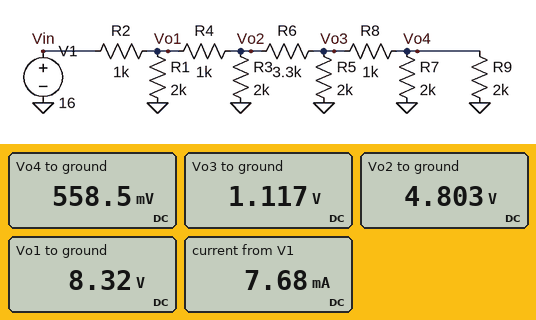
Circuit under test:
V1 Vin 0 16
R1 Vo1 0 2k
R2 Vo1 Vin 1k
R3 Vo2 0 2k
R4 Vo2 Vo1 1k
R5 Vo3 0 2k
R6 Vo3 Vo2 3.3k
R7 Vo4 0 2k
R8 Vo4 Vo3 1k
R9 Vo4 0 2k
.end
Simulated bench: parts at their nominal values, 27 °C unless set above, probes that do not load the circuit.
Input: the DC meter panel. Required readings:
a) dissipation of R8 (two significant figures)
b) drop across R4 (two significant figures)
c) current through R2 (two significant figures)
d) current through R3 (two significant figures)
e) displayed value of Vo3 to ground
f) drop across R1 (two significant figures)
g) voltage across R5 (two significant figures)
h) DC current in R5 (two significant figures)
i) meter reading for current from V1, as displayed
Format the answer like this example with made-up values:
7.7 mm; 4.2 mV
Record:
310 µW; 3.5 V; 7.7 mA; 2.4 mA; 1.117 V; 8.3 V; 1.1 V; 560 µA; 7.68 mA
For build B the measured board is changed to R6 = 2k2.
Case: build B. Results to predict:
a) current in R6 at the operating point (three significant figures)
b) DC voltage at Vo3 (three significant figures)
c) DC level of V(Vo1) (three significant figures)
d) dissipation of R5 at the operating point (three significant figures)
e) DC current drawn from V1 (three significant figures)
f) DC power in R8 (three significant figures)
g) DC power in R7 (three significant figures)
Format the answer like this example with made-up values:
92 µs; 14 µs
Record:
1.42 mA; 1.42 V; 8.21 V; 1.00 mW; 7.79 mA; 501 µW; 251 µW
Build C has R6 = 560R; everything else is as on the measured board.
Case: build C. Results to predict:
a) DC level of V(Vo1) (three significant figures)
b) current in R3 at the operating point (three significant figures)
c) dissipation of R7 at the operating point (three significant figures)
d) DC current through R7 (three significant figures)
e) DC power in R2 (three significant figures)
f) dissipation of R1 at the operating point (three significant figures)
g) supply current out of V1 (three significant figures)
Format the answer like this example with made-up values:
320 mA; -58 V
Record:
7.87 V; 1.84 mA; 694 µW; 589 µA; 66.1 mW; 31.0 mW; 8.13 mA
